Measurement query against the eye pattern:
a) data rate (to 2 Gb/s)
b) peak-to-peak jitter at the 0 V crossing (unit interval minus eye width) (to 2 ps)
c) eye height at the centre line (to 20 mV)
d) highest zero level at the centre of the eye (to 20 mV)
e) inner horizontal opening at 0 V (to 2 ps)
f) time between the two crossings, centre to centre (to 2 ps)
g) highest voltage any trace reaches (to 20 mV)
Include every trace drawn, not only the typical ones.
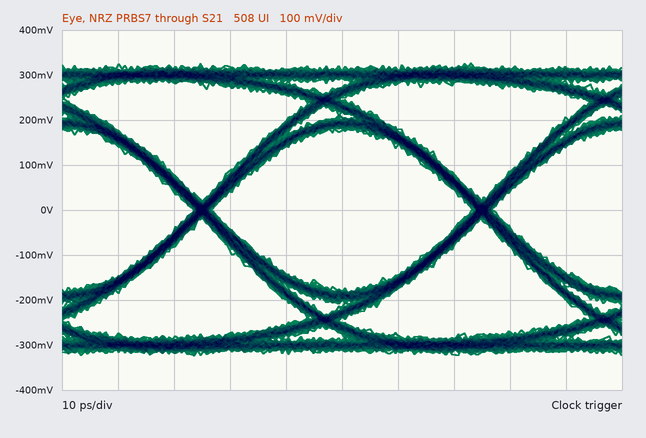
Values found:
20 Gb/s
4 ps
360 mV
-180 mV
46 ps
50 ps
320 mV
